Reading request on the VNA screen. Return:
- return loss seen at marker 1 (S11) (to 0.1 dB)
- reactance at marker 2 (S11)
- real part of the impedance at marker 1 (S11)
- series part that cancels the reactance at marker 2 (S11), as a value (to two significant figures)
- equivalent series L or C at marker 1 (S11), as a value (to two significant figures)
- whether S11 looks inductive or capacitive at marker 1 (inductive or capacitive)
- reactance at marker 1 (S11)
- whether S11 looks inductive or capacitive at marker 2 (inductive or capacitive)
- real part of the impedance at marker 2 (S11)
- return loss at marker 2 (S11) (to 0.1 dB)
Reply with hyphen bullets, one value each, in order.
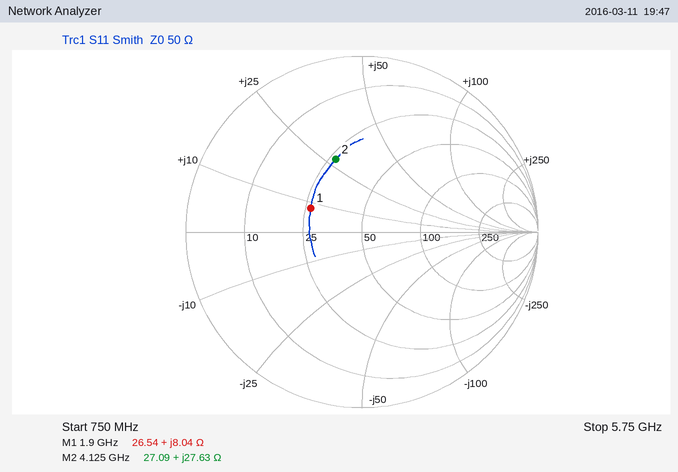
- 9.8 dB
- +27.63 Ω
- 26.54 Ω
- 1.4 pF
- 670 pH
- inductive
- +8.04 Ω
- inductive
- 27.09 Ω
- 7.2 dB
